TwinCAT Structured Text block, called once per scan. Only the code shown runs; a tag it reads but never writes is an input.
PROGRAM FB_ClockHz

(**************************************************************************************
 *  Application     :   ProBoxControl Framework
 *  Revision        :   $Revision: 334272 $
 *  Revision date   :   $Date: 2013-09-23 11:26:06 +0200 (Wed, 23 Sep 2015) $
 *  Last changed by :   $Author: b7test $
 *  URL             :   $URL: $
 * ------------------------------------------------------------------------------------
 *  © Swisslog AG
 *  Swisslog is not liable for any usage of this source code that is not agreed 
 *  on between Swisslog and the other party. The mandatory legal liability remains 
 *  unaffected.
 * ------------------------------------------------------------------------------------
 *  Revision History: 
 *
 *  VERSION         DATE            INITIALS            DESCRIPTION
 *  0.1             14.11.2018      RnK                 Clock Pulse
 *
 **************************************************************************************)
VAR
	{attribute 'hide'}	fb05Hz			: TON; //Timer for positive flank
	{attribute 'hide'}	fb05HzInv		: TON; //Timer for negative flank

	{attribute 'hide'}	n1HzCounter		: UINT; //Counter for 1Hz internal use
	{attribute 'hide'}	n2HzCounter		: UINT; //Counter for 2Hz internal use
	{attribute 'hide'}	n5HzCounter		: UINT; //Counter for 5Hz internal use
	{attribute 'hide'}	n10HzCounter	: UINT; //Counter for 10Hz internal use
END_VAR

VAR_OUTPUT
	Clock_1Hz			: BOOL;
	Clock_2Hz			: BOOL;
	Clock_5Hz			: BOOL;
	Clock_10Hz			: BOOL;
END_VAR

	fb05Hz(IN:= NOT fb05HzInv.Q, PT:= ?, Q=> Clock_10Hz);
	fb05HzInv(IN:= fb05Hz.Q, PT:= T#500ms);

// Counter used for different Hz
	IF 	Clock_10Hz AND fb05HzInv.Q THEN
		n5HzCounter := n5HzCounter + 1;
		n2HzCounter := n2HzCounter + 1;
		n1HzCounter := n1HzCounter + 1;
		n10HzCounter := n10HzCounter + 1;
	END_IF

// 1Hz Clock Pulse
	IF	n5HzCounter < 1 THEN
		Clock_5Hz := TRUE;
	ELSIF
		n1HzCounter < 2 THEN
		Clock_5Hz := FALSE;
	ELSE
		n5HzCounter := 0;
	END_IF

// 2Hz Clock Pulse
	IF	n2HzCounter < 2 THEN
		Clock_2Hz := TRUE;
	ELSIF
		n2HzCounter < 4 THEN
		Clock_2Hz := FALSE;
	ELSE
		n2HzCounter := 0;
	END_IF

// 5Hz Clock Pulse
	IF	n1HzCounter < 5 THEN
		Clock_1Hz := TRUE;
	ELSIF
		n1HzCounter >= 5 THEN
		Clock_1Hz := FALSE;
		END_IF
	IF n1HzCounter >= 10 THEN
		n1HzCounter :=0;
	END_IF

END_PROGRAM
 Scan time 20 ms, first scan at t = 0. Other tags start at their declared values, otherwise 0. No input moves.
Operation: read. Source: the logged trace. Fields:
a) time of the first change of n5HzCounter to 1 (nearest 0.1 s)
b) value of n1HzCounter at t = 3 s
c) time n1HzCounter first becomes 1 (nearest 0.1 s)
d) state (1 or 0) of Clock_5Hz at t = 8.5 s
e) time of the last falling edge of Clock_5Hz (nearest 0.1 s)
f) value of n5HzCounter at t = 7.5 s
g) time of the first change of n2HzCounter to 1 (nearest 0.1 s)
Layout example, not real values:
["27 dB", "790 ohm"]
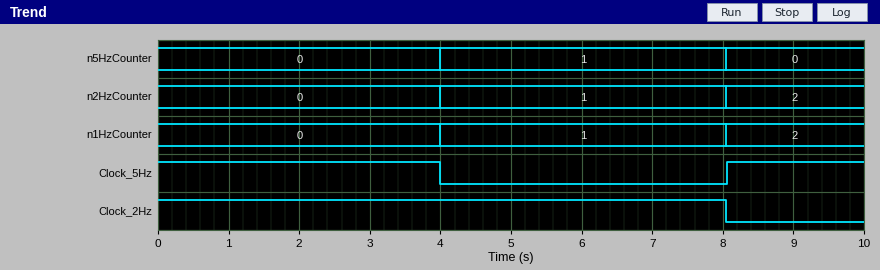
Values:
["4.0 s", "0", "4.0 s", "1", "4.0 s", "1", "4.0 s"]
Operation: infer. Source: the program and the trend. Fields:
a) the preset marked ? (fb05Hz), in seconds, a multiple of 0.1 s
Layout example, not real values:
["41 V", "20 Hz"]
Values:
["3.5 s"]
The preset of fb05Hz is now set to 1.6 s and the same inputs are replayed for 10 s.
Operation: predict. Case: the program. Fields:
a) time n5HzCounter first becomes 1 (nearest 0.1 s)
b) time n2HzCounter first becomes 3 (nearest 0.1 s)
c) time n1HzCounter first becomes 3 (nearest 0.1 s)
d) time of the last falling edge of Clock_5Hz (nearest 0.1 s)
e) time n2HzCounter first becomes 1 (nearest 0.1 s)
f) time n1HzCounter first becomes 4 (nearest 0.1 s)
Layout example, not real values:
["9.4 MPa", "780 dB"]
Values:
["2.1 s", "6.4 s", "6.4 s", "2.1 s", "2.1 s", "8.5 s"]
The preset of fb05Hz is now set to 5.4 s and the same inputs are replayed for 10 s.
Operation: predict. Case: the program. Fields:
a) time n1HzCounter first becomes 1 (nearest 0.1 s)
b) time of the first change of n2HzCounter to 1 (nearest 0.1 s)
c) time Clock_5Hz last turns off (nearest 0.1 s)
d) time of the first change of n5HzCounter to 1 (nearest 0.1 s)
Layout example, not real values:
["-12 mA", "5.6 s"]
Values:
["5.9 s", "5.9 s", "5.9 s", "5.9 s"]
